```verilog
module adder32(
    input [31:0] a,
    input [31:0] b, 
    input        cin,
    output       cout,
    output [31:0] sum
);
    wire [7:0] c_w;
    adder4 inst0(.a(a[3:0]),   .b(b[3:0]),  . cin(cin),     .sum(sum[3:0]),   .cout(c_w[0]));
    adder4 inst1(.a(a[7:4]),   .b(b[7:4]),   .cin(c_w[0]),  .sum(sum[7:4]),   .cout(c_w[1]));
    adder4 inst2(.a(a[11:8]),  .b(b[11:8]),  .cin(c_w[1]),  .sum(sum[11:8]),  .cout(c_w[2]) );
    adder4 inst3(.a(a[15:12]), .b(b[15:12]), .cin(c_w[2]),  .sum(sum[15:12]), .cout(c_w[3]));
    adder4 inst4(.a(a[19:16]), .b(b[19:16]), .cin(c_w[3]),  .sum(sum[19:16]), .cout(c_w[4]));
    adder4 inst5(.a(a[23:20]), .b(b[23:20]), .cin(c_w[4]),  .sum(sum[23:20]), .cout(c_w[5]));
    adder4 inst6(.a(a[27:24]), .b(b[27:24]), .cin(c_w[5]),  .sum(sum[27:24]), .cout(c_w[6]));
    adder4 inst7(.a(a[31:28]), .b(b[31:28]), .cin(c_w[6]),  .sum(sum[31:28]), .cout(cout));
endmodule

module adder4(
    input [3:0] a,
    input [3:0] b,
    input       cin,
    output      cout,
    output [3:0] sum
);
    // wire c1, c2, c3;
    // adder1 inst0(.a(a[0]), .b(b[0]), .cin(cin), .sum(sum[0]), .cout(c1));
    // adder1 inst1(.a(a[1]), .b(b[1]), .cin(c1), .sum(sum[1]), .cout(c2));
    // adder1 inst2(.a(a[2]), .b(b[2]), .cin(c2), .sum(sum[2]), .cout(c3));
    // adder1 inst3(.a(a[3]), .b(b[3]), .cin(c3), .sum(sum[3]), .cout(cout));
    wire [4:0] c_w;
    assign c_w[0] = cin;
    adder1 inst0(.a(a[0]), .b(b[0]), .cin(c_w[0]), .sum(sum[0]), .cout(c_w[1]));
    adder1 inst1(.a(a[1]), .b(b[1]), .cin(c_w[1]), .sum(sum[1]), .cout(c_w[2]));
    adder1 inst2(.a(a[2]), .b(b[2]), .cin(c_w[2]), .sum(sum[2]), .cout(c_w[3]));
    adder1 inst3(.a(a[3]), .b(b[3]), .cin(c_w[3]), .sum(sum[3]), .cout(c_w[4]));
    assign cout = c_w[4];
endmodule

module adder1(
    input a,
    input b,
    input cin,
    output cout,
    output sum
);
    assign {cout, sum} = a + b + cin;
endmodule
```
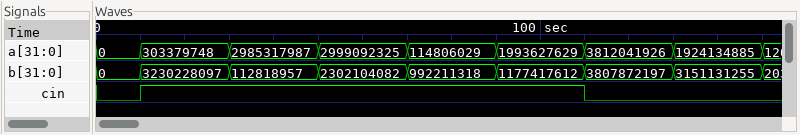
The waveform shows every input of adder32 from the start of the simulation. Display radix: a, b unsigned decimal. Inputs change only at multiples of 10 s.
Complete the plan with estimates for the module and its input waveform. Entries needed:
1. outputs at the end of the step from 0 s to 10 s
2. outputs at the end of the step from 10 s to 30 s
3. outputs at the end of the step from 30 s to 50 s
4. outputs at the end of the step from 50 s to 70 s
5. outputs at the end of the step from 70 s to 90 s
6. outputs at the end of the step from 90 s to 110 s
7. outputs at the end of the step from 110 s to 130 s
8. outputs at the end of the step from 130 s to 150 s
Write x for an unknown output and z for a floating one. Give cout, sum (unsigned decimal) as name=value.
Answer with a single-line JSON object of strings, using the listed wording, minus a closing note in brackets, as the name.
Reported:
{"outputs at the end of the step from 0 s to 10 s": "cout=0, sum=0", "outputs at the end of the step from 10 s to 30 s": "cout=0, sum=3533607846", "outputs at the end of the step from 30 s to 50 s": "cout=0, sum=3098136945", "outputs at the end of the step from 50 s to 70 s": "cout=1, sum=1006229112", "outputs at the end of the step from 70 s to 90 s": "cout=0, sum=1107017348", "outputs at the end of the step from 90 s to 110 s": "cout=0, sum=3171045242", "outputs at the end of the step from 110 s to 130 s": "cout=1, sum=3324946827", "outputs at the end of the step from 130 s to 150 s": "cout=1, sum=780298844"}
